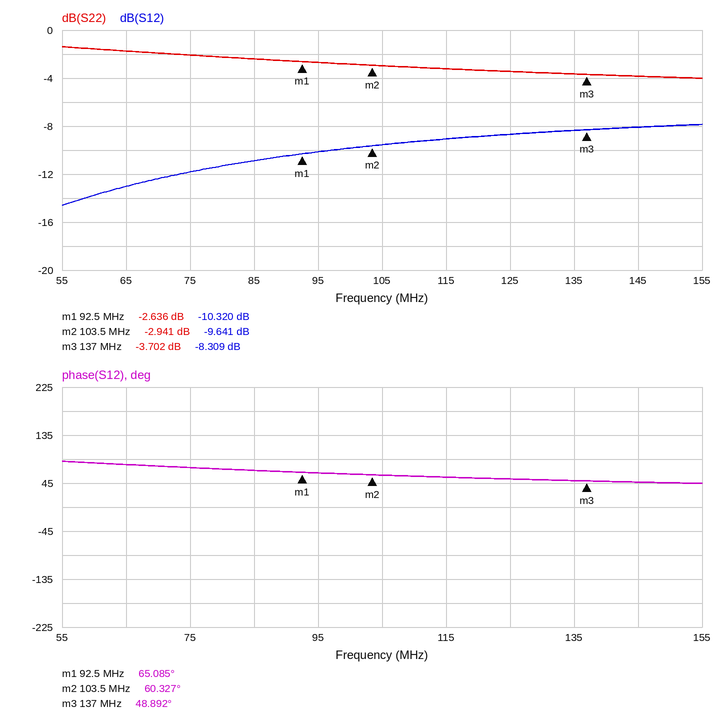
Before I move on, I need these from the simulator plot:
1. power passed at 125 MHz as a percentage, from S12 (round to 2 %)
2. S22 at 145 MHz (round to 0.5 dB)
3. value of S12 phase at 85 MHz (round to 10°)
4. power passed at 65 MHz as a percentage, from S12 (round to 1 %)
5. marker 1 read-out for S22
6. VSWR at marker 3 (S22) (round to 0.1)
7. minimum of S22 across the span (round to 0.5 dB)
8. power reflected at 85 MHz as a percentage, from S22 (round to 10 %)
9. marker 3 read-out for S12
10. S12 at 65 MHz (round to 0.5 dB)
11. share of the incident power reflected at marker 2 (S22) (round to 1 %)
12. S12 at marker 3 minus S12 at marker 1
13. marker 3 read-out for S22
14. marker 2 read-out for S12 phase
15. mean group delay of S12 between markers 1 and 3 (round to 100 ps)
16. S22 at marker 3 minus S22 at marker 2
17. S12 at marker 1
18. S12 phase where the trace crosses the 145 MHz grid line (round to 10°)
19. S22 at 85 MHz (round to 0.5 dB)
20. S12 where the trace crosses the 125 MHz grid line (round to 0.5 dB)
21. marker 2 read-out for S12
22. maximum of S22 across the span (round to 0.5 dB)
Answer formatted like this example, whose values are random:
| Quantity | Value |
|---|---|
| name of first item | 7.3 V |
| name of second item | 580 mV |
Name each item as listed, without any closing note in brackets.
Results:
| Quantity | Value |
|---|---|
| power passed at 125 MHz as a percentage, from S12 | 14 % |
| S22 at 145 MHz | -4.0 dB |
| value of S12 phase at 85 MHz | 70° |
| power passed at 65 MHz as a percentage, from S12 | 5 % |
| marker 1 read-out for S22 | -2.636 dB |
| VSWR at marker 3 (S22) | 4.8 |
| minimum of S22 across the span | -4.0 dB |
| power reflected at 85 MHz as a percentage, from S22 | 60 % |
| marker 3 read-out for S12 | -8.309 dB |
| S12 at 65 MHz | -13.0 dB |
| share of the incident power reflected at marker 2 (S22) | 51 % |
| S12 at marker 3 minus S12 at marker 1 | 2.011 dB |
| marker 3 read-out for S22 | -3.702 dB |
| marker 2 read-out for S12 phase | 60.327° |
| mean group delay of S12 between markers 1 and 3 | 1.0 ns |
| S22 at marker 3 minus S22 at marker 2 | -0.761 dB |
| S12 at marker 1 | -10.320 dB |
| S12 phase where the trace crosses the 145 MHz grid line | 50° |
| S22 at 85 MHz | -2.5 dB |
| S12 where the trace crosses the 125 MHz grid line | -8.5 dB |
| marker 2 read-out for S12 | -9.641 dB |
| maximum of S22 across the span | -1.5 dB |
